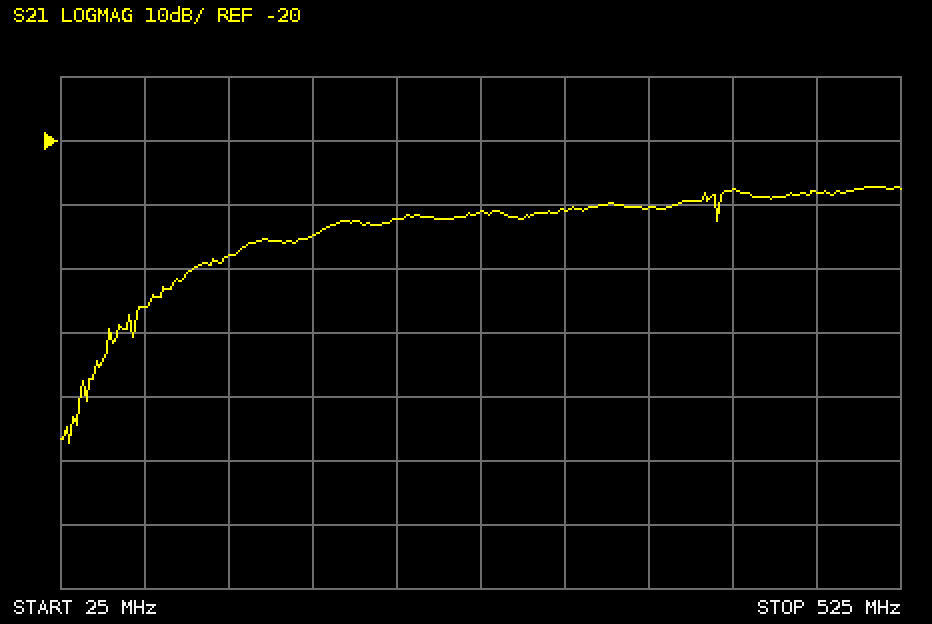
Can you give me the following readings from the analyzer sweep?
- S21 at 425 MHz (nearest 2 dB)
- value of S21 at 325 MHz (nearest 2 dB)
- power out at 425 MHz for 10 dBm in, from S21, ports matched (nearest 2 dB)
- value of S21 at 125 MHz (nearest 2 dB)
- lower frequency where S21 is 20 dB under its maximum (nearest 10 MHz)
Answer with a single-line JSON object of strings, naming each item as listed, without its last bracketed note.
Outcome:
{"S21 at 425 MHz": "-28 dB", "value of S21 at 325 MHz": "-30 dB", "power out at 425 MHz for 10 dBm in, from S21, ports matched": "-18 dBm", "value of S21 at 125 MHz": "-38 dB", "lower frequency where S21 is 20 dB under its maximum": "70 MHz"}
